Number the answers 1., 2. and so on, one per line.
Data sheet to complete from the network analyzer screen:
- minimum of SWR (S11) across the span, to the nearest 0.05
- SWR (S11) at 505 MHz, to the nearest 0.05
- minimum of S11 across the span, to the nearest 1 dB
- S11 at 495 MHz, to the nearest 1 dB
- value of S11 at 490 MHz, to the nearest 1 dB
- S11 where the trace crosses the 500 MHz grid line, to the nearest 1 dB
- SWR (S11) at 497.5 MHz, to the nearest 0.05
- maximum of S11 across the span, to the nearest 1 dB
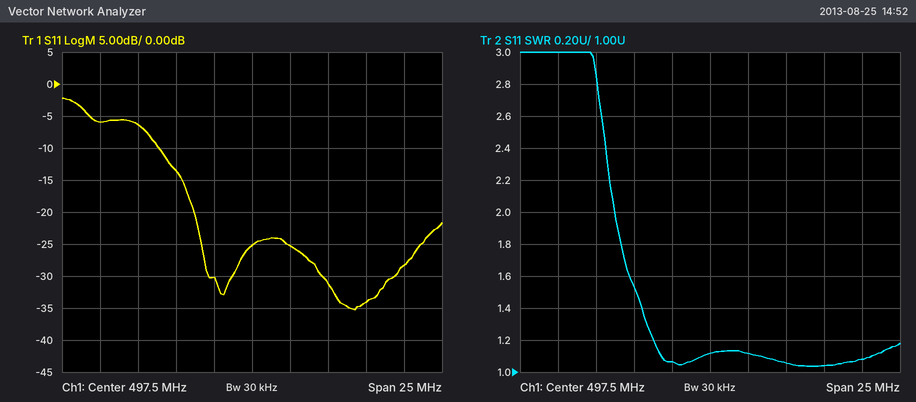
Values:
1. 1.05
2. 1.05
3. -35 dB
4. -30 dB
5. -6 dB
6. -25 dB
7. 1.10
8. -2 dB
